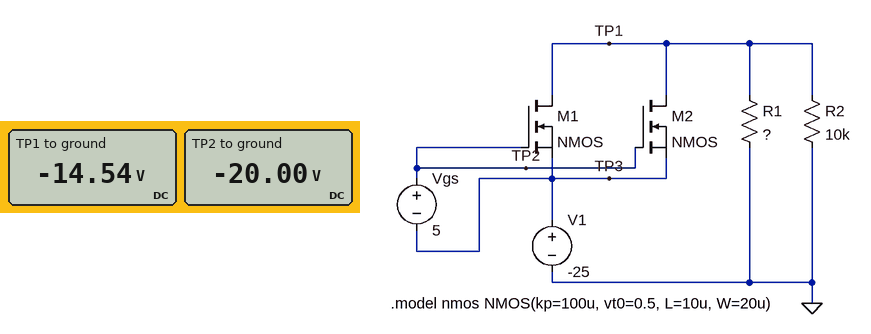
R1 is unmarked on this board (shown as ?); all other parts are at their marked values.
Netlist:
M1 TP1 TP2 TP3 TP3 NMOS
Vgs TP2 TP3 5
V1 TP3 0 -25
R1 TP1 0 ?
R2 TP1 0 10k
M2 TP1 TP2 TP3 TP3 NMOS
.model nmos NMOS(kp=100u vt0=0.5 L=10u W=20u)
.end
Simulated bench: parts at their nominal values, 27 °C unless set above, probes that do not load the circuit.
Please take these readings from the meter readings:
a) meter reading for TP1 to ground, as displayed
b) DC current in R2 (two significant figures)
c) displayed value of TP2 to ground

-14.54 V
1.5 mA
-20.00 V
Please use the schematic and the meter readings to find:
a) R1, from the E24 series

5.6 kΩ
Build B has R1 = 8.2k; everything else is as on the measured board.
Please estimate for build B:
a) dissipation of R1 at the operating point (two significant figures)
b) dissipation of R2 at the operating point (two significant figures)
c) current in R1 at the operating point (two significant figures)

41 mW
33 mW
2.2 mA
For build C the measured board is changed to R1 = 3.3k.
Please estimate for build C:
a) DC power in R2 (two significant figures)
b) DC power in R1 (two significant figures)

10 mW
31 mW
